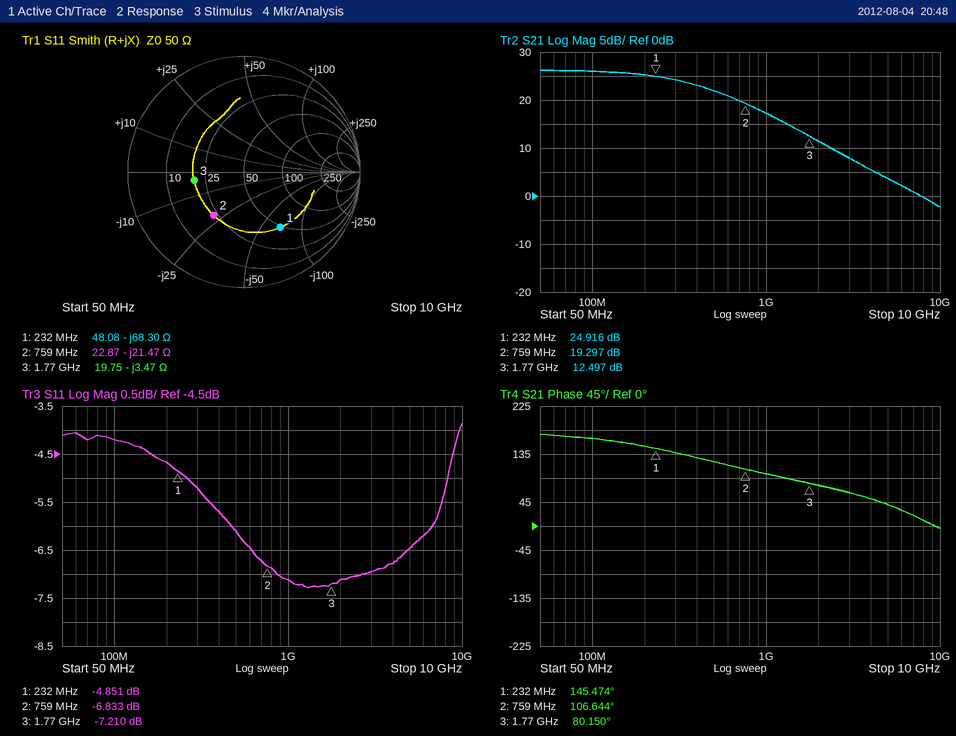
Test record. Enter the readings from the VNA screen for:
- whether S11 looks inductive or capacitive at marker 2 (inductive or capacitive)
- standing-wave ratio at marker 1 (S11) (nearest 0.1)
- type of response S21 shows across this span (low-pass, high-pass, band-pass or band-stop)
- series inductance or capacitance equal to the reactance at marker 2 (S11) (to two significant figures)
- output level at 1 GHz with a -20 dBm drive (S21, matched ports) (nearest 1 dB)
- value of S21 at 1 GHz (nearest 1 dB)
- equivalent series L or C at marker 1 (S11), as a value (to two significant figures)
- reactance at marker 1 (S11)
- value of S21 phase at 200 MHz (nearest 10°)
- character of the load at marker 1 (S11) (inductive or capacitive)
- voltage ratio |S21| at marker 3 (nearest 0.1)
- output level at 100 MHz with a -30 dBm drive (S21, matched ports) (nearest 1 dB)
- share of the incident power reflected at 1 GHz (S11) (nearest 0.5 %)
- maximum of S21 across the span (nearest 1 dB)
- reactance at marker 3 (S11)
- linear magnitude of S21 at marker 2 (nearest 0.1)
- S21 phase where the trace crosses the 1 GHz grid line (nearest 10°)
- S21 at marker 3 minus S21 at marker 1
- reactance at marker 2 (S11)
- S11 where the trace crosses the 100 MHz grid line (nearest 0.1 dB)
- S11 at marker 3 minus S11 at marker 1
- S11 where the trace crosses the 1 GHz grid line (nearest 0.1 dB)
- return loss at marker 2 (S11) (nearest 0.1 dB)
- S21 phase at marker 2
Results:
capacitive
3.7
low-pass
9.8 pF
-3 dBm
17 dB
10 pF
-68.30 Ω
150°
capacitive
4.2
-4 dBm
19.5 %
26 dB
-3.47 Ω
9.2
100°
-12.419 dB
-21.47 Ω
-4.2 dB
-2.359 dB
-7.1 dB
6.8 dB
106.644°
